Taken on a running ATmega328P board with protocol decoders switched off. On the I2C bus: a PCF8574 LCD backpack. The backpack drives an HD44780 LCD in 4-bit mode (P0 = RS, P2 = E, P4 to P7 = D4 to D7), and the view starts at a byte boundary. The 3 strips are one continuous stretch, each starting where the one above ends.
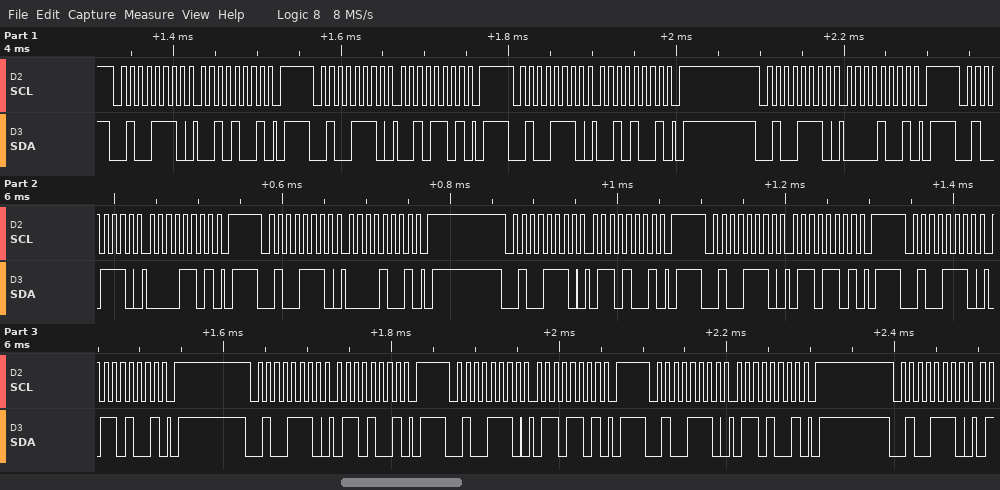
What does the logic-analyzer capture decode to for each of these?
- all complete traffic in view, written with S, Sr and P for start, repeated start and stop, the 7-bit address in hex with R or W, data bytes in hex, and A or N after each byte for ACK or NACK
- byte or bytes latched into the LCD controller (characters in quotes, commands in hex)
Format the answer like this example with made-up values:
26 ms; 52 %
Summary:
S 27W A 29 A P S 27W A 2D A P S 27W A 29 A P S 27W A 09 A P S 27W A 0D A P S 27W A 09 A P S 27W A 69 A P S 27W A 6D A P S 27W A 69 A P S 27W A 69 A P S 27W A 6D A P S 27W A 69 A P S 27W A; ' ' 'f'
